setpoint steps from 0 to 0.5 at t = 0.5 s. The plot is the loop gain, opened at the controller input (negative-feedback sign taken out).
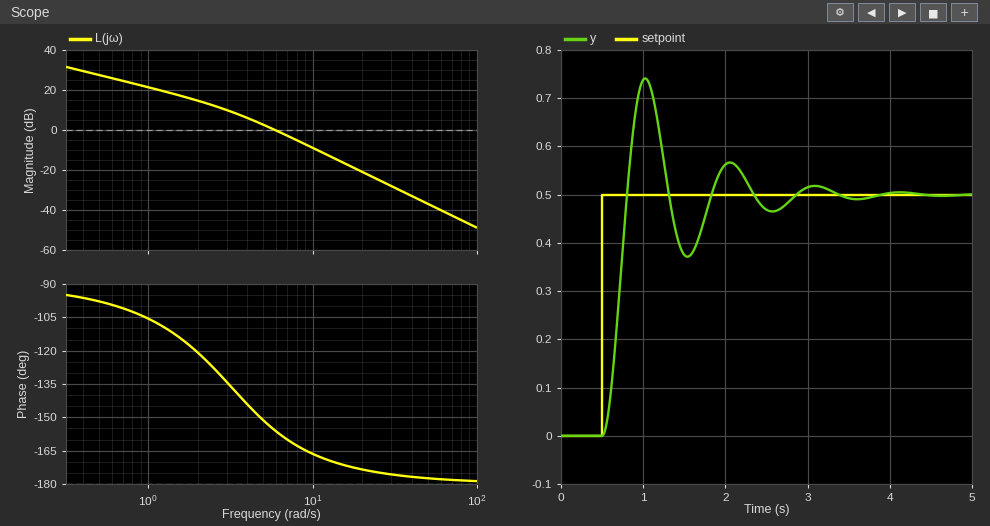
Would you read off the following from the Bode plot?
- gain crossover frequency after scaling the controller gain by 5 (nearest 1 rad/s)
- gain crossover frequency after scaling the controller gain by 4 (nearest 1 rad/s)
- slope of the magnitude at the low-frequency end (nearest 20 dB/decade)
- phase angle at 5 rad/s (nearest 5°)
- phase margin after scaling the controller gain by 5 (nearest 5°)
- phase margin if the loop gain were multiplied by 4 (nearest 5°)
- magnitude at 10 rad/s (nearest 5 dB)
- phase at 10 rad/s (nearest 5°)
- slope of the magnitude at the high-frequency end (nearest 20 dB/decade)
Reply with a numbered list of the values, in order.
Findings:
1. 13 rad/s
2. 12 rad/s
3. -20 dB/decade
4. -150°
5. 10°
6. 10°
7. -10 dB
8. -165°
9. -40 dB/decade
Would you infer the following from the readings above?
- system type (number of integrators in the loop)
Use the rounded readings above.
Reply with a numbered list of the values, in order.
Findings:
1. 1
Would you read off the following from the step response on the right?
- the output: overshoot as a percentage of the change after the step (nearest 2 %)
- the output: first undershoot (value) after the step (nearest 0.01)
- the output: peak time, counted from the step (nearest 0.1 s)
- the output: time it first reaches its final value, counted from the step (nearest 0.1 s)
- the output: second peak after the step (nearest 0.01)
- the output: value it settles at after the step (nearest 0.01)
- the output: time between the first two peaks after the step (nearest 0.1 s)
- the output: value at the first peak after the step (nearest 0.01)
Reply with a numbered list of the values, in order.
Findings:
1. 48 %
2. 0.37
3. 0.5 s
4. 0.3 s
5. 0.57
6. 0.50
7. 1.0 s
8. 0.74
